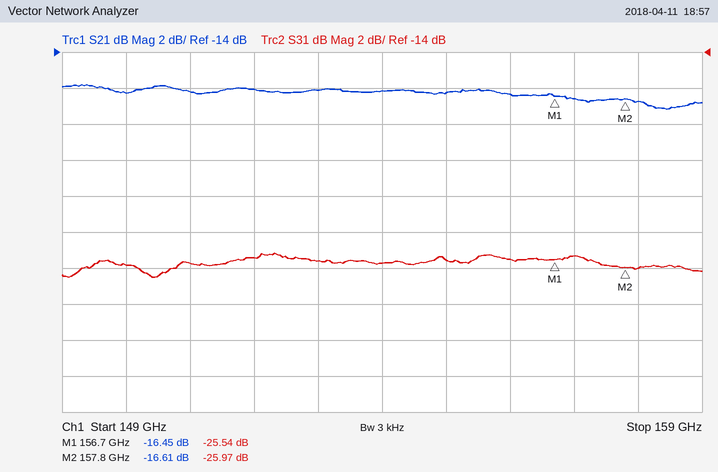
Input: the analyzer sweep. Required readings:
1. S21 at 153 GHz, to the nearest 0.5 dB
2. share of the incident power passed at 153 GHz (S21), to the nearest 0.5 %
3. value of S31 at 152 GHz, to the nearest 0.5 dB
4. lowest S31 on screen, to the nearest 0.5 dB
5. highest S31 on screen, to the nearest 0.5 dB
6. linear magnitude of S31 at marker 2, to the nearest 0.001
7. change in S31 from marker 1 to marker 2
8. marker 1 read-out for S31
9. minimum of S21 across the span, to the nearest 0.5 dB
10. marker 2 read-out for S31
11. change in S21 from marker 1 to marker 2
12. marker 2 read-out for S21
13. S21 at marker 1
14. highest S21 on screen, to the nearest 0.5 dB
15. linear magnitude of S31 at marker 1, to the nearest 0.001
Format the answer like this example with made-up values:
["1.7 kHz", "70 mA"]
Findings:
["-16.0 dB", "2.5 %", "-25.5 dB", "-26.5 dB", "-25.0 dB", "0.050", "-0.43 dB", "-25.54 dB", "-17.0 dB", "-25.97 dB", "-0.16 dB", "-16.61 dB", "-16.45 dB", "-16.0 dB", "0.053"]
